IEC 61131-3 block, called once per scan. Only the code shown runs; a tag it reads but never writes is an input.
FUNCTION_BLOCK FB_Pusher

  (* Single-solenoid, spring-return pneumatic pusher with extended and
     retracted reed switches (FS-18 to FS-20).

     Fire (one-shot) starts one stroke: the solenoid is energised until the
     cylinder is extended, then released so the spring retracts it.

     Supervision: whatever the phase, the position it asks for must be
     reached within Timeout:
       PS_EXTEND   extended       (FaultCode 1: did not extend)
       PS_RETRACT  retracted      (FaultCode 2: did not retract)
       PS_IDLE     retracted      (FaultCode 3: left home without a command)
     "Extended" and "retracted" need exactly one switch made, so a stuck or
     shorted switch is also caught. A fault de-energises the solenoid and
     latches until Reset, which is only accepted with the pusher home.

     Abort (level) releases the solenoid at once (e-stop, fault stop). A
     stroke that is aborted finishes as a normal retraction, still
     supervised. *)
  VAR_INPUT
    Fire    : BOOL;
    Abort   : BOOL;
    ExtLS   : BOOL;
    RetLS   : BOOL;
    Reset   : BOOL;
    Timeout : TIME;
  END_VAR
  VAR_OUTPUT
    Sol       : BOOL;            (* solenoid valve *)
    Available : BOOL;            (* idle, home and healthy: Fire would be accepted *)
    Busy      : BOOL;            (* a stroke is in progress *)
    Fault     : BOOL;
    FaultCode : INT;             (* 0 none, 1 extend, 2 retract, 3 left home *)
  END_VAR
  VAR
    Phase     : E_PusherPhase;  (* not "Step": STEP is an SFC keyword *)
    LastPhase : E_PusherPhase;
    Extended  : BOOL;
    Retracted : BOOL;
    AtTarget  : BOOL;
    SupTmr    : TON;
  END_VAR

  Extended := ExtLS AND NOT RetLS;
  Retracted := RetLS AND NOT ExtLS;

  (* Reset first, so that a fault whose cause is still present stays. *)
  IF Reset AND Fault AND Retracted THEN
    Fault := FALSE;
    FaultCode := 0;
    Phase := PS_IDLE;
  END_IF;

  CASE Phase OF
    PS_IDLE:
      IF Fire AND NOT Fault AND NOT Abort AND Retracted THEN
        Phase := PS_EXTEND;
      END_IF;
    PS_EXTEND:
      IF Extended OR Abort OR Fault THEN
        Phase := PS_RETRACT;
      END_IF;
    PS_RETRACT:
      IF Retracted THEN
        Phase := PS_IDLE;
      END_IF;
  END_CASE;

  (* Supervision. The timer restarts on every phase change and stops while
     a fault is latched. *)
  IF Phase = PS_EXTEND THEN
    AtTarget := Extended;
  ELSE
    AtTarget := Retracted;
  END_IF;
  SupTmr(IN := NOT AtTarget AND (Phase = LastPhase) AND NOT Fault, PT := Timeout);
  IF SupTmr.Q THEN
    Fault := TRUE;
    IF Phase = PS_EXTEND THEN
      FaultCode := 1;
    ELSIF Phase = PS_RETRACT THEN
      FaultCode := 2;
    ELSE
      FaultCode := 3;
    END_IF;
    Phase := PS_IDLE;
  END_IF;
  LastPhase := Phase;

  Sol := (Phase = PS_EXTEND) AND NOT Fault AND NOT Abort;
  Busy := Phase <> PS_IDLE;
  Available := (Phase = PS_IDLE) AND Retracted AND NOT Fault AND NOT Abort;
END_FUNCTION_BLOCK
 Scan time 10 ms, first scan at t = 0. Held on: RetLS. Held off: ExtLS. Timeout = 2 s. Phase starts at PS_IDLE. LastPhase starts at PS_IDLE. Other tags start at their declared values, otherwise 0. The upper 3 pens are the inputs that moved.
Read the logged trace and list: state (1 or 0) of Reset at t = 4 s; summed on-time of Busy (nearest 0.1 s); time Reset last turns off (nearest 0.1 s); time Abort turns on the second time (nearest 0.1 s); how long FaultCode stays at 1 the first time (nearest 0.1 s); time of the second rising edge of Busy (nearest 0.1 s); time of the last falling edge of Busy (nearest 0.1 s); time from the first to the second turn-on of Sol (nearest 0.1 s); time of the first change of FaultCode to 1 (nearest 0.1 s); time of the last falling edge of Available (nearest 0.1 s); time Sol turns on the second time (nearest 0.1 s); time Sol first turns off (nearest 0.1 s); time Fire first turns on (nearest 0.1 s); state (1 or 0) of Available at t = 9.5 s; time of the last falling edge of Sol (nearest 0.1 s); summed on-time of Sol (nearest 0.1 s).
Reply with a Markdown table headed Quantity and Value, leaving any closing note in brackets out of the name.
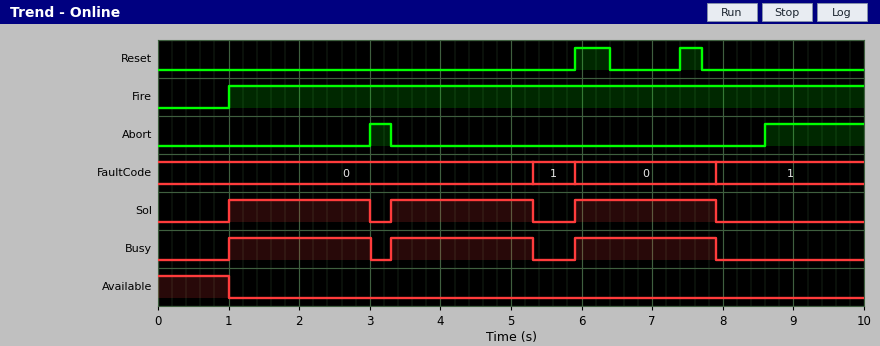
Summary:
| Quantity | Value |
|---|---|
| state (1 or 0) of Reset at t = 4 s | 0 |
| summed on-time of Busy | 6.0 s |
| time Reset last turns off | 7.7 s |
| time Abort turns on the second time | 8.6 s |
| how long FaultCode stays at 1 the first time | 0.6 s |
| time of the second rising edge of Busy | 3.3 s |
| time of the last falling edge of Busy | 7.9 s |
| time from the first to the second turn-on of Sol | 2.3 s |
| time of the first change of FaultCode to 1 | 5.3 s |
| time of the last falling edge of Available | 1.0 s |
| time Sol turns on the second time | 3.3 s |
| time Sol first turns off | 3.0 s |
| time Fire first turns on | 1.0 s |
| state (1 or 0) of Available at t = 9.5 s | 0 |
| time of the last falling edge of Sol | 7.9 s |
| summed on-time of Sol | 6.0 s |
